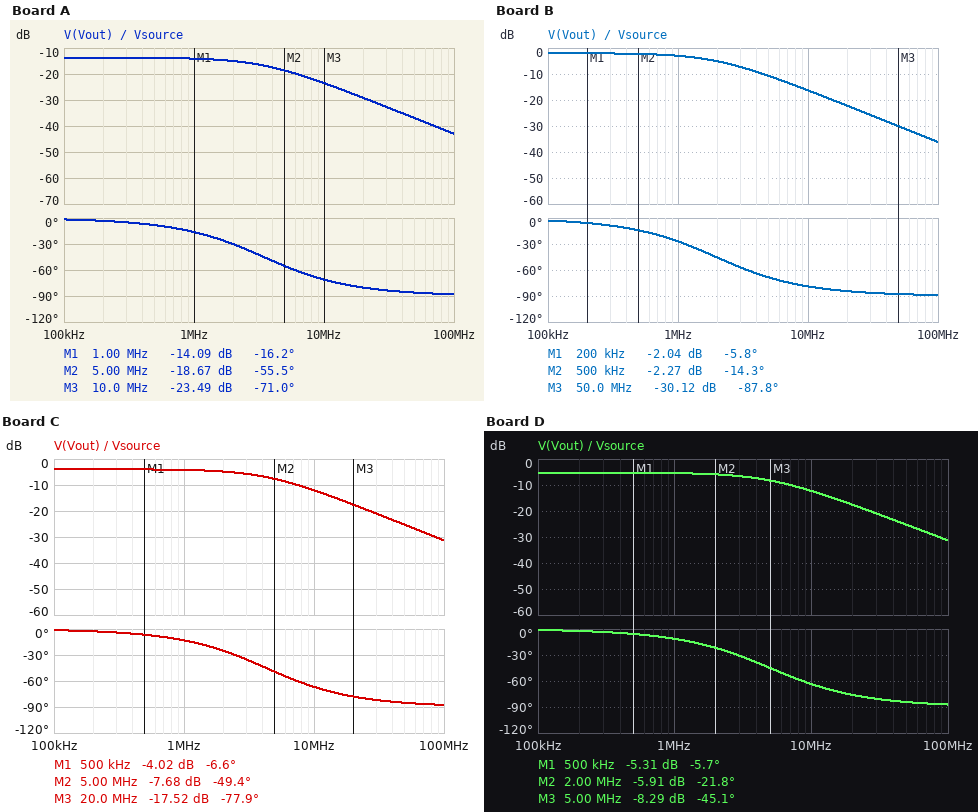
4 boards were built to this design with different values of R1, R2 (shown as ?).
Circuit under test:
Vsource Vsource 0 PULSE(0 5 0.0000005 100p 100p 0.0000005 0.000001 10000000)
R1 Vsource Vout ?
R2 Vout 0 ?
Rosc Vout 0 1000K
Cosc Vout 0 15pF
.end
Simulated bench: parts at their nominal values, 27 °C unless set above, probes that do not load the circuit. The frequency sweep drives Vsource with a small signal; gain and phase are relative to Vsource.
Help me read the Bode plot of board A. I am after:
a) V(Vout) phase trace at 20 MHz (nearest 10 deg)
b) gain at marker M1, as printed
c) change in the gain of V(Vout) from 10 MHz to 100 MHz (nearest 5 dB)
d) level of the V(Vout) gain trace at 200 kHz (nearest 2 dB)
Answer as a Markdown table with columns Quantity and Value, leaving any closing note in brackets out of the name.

| Quantity | Value |
|---|---|
| V(Vout) phase trace at 20 MHz | -80 deg |
| gain at marker M1, as printed | -14.09 dB |
| change in the gain of V(Vout) from 10 MHz to 100 MHz | -20 dB |
| level of the V(Vout) gain trace at 200 kHz | -14 dB |
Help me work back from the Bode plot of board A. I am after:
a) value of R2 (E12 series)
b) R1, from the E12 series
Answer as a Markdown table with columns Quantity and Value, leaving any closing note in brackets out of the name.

| Quantity | Value |
|---|---|
| value of R2 | 3.9 kΩ |
| R1, from the E12 series | 15 kΩ |
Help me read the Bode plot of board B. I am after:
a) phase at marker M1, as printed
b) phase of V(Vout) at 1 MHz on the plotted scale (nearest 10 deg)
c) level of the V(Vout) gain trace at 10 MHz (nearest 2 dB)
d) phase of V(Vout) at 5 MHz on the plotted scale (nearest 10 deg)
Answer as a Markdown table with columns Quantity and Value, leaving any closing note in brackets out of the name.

| Quantity | Value |
|---|---|
| phase at marker M1, as printed | -5.8 deg |
| phase of V(Vout) at 1 MHz on the plotted scale | -30 deg |
| level of the V(Vout) gain trace at 10 MHz | -16 dB |
| phase of V(Vout) at 5 MHz on the plotted scale | -70 deg |
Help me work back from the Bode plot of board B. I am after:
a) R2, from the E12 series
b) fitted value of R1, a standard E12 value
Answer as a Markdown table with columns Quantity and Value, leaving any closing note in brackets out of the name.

| Quantity | Value |
|---|---|
| R2, from the E12 series | 27 kΩ |
| fitted value of R1, a standard E12 value | 6.8 kΩ |
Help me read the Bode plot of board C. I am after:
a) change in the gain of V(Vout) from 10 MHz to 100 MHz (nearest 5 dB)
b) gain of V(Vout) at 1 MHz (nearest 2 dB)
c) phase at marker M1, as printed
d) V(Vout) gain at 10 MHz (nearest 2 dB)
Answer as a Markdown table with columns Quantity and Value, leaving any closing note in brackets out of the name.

| Quantity | Value |
|---|---|
| change in the gain of V(Vout) from 10 MHz to 100 MHz | -20 dB |
| gain of V(Vout) at 1 MHz | -4 dB |
| phase at marker M1, as printed | -6.6 deg |
| V(Vout) gain at 10 MHz | -12 dB |
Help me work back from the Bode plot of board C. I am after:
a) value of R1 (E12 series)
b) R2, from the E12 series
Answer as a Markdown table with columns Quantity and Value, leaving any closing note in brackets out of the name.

| Quantity | Value |
|---|---|
| value of R1 | 3.9 kΩ |
| R2, from the E12 series | 6.8 kΩ |
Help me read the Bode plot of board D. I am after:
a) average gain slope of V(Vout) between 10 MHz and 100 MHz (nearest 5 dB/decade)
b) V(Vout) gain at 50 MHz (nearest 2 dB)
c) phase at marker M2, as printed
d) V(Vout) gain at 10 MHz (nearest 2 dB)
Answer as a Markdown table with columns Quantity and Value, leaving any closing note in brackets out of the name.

| Quantity | Value |
|---|---|
| average gain slope of V(Vout) between 10 MHz and 100 MHz | -20 dB/decade |
| V(Vout) gain at 50 MHz | -26 dB |
| phase at marker M2, as printed | -21.8 deg |
| V(Vout) gain at 10 MHz | -12 dB |
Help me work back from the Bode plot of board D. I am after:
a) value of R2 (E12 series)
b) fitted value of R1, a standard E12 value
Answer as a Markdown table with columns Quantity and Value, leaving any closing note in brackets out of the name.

| Quantity | Value |
|---|---|
| value of R2 | 4.7 kΩ |
| fitted value of R1, a standard E12 value | 3.9 kΩ |
